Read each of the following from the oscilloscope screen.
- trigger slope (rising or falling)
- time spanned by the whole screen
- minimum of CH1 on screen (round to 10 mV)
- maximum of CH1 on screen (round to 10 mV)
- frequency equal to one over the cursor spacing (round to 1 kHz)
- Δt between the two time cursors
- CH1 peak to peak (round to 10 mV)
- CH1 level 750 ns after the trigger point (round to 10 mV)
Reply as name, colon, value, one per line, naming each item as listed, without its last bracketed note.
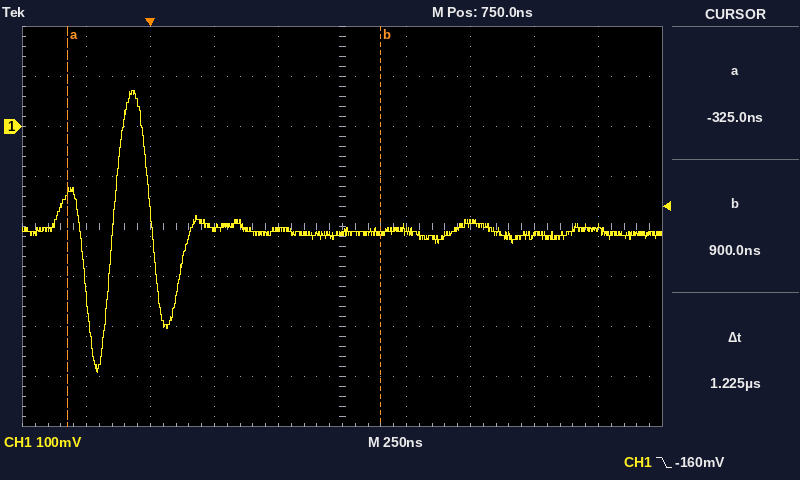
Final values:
trigger slope: falling
time spanned by the whole screen: 2.5 µs
minimum of CH1 on screen: -490 mV
maximum of CH1 on screen: 70 mV
frequency equal to one over the cursor spacing: 816 kHz
Δt between the two time cursors: 1.225 µs
CH1 peak to peak: 560 mV
CH1 level 750 ns after the trigger point: -210 mV
